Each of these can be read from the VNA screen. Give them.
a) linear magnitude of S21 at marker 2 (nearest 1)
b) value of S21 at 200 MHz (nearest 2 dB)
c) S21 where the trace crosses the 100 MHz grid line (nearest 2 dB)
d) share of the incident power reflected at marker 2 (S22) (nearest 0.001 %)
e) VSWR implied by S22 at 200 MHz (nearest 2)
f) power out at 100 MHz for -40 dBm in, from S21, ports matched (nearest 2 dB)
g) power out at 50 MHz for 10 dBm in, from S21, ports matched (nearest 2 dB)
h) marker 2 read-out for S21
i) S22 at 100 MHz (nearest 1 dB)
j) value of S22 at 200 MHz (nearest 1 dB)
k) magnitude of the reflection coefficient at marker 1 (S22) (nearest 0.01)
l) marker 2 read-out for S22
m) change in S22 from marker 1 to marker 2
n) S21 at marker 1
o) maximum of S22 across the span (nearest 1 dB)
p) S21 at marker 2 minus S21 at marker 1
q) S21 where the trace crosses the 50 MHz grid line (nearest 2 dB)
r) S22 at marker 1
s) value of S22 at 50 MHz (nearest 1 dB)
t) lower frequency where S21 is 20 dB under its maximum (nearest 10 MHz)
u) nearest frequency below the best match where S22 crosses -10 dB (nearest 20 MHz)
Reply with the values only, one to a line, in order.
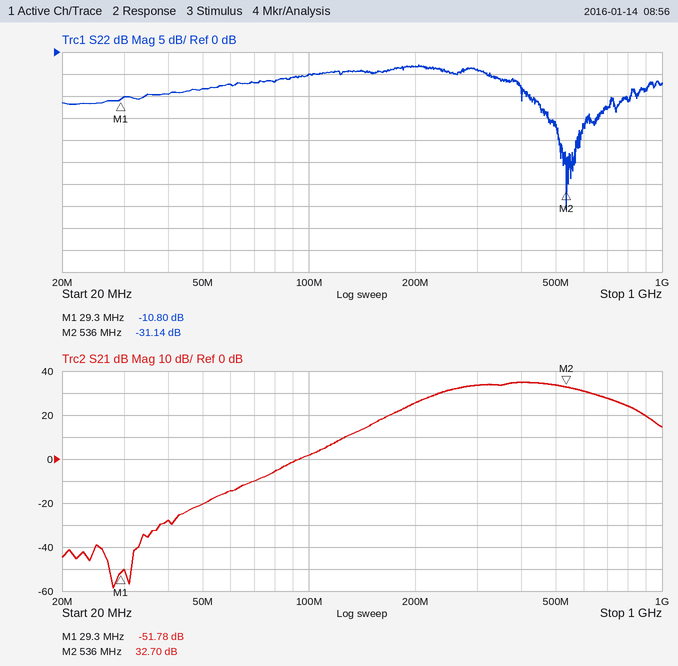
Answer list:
43
26 dB
2 dB
0.077 %
6
-38 dBm
-10 dBm
32.70 dB
-5 dB
-3 dB
0.29
-31.14 dB
-20.34 dB
-51.78 dB
-3 dB
84.48 dB
-20 dB
-10.80 dB
-8 dB
150 MHz
420 MHz
